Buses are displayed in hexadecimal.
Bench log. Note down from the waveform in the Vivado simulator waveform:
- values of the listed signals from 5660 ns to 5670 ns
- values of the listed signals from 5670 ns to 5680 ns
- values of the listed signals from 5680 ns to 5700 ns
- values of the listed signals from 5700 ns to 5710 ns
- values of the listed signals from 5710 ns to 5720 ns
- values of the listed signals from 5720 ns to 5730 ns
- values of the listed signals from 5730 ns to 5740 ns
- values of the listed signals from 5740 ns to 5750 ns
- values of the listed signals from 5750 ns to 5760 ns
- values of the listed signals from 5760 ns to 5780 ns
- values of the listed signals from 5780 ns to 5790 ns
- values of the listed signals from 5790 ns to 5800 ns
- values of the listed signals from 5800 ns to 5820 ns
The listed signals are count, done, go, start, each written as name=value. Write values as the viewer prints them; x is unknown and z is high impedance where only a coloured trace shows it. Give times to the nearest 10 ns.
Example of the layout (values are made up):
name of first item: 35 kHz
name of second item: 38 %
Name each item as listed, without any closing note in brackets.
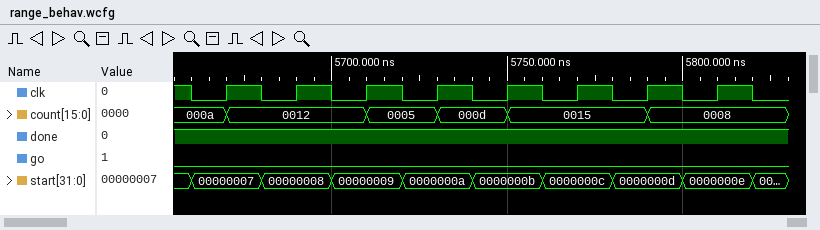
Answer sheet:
values of the listed signals from 5660 ns to 5670 ns: count=000a, done=1, go=0, start=00000007
values of the listed signals from 5670 ns to 5680 ns: count=0012, done=1, go=0, start=00000007
values of the listed signals from 5680 ns to 5700 ns: count=0012, done=1, go=0, start=00000008
values of the listed signals from 5700 ns to 5710 ns: count=0012, done=1, go=0, start=00000009
values of the listed signals from 5710 ns to 5720 ns: count=0005, done=1, go=0, start=00000009
values of the listed signals from 5720 ns to 5730 ns: count=0005, done=1, go=0, start=0000000a
values of the listed signals from 5730 ns to 5740 ns: count=000d, done=1, go=0, start=0000000a
values of the listed signals from 5740 ns to 5750 ns: count=000d, done=1, go=0, start=0000000b
values of the listed signals from 5750 ns to 5760 ns: count=0015, done=1, go=0, start=0000000b
values of the listed signals from 5760 ns to 5780 ns: count=0015, done=1, go=0, start=0000000c
values of the listed signals from 5780 ns to 5790 ns: count=0015, done=1, go=0, start=0000000d
values of the listed signals from 5790 ns to 5800 ns: count=0008, done=1, go=0, start=0000000d
values of the listed signals from 5800 ns to 5820 ns: count=0008, done=1, go=0, start=0000000e
